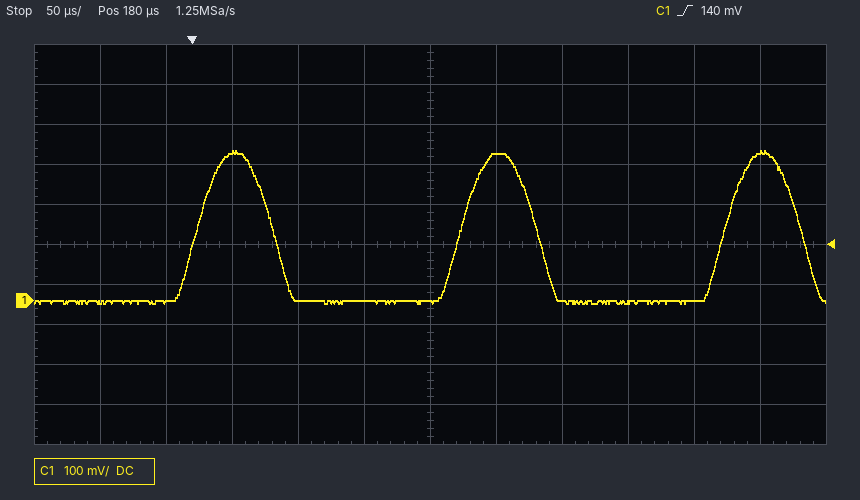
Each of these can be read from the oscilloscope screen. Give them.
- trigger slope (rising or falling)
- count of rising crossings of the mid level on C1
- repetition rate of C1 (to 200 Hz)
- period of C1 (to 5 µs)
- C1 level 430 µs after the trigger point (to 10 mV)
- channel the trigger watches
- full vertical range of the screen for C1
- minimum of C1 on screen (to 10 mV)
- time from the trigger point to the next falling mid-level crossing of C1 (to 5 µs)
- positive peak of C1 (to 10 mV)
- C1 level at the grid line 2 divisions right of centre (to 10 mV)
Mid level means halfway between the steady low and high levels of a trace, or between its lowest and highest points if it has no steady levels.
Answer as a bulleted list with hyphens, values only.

- rising
- 3
- 5.0 kHz
- 200 µs
- 370 mV
- C1
- 1 V
- -10 mV
- 60 µs
- 380 mV
- 0 mV
